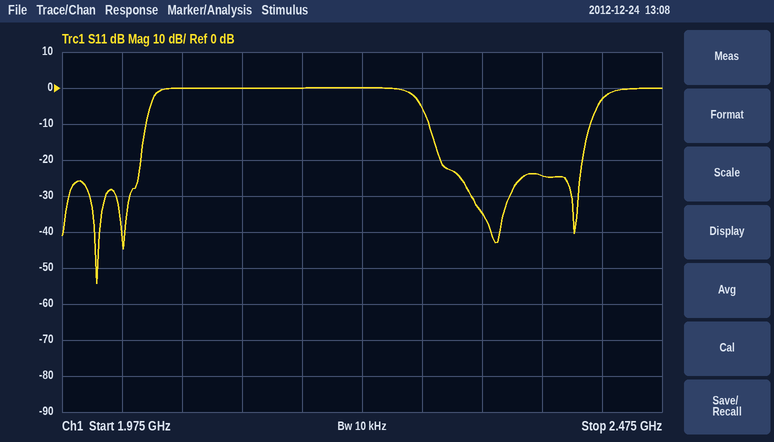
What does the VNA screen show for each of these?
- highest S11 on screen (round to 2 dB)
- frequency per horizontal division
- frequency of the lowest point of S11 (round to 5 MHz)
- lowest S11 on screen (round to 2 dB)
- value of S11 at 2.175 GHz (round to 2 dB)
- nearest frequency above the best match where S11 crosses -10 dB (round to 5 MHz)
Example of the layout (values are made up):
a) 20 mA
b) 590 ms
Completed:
a) 0 dB
b) 50 MHz
c) 2.005 GHz
d) -54 dB
e) 0 dB
f) 2.045 GHz
